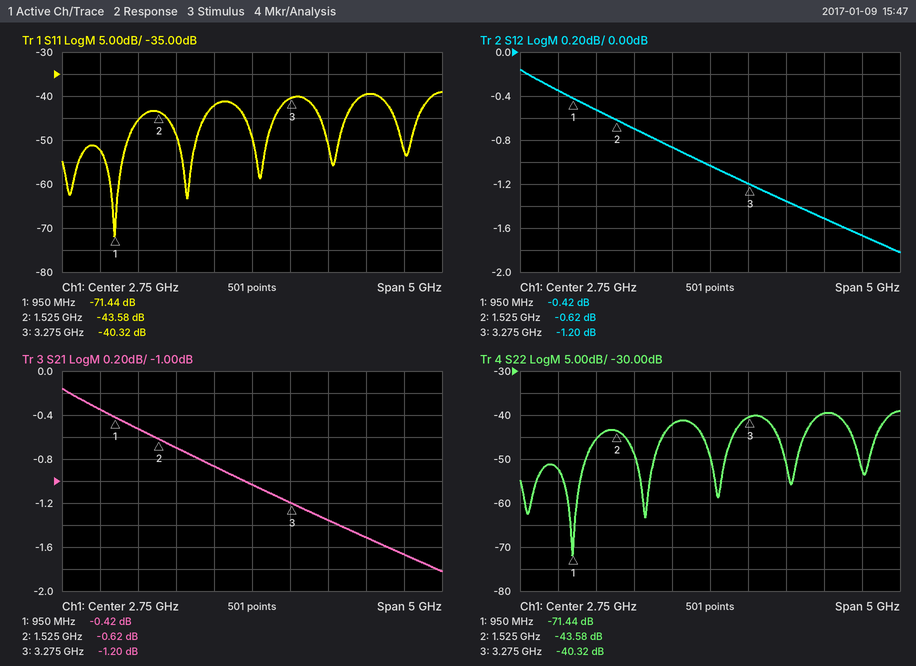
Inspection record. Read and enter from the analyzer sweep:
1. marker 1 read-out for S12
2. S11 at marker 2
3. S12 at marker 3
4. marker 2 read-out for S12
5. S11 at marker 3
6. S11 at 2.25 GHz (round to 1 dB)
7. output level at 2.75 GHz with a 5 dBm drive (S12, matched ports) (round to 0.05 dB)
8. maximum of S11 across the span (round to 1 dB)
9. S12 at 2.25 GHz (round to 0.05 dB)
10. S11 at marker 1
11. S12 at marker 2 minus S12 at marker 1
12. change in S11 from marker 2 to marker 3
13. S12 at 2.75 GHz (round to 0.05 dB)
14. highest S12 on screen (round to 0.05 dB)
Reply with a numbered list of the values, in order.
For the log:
1. -0.42 dB
2. -43.58 dB
3. -1.20 dB
4. -0.62 dB
5. -40.32 dB
6. -42 dB
7. 3.95 dBm
8. -39 dB
9. -0.85 dB
10. -71.44 dB
11. -0.20 dB
12. 3.26 dB
13. -1.05 dB
14. -0.15 dB
